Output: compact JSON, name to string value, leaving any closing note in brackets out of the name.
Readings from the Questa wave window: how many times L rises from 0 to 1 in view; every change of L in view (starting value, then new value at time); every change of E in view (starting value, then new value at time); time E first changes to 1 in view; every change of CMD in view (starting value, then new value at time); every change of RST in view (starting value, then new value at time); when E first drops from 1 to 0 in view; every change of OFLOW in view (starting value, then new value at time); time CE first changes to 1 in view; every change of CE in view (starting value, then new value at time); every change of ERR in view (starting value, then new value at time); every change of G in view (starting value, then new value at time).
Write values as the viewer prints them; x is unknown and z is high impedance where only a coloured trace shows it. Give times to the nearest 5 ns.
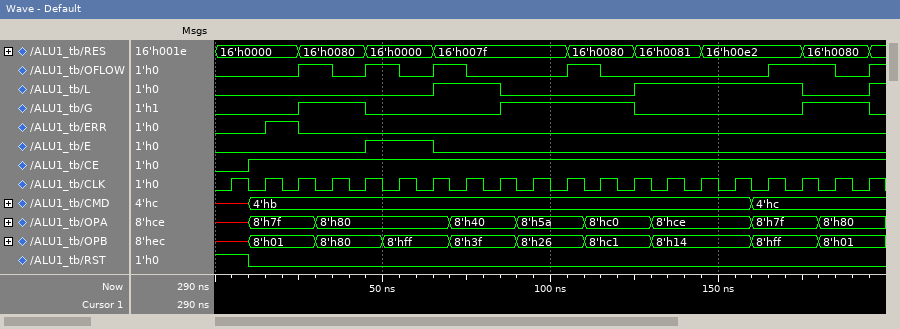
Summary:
{"how many times L rises from 0 to 1 in view": "3", "every change of L in view": "0, 1 at 65 ns, 0 at 85 ns, 1 at 125 ns, 0 at 175 ns, 1 at 195 ns", "every change of E in view": "0, 1 at 45 ns, 0 at 65 ns", "time E first changes to 1 in view": "45 ns", "every change of CMD in view": "x, 4'hb at 10 ns, 4'hc at 160 ns", "every change of RST in view": "1, 0 at 10 ns", "when E first drops from 1 to 0 in view": "65 ns", "every change of OFLOW in view": "0, 1 at 25 ns, 0 at 35 ns, 1 at 45 ns, 0 at 55 ns, 1 at 65 ns, 0 at 75 ns, 1 at 105 ns, 0 at 115 ns, 1 at 165 ns, 0 at 185 ns, 1 at 195 ns", "time CE first changes to 1 in view": "10 ns", "every change of CE in view": "0, 1 at 10 ns", "every change of ERR in view": "0, 1 at 15 ns, 0 at 25 ns", "every change of G in view": "0, 1 at 25 ns, 0 at 45 ns, 1 at 85 ns, 0 at 125 ns, 1 at 175 ns, 0 at 195 ns"}
